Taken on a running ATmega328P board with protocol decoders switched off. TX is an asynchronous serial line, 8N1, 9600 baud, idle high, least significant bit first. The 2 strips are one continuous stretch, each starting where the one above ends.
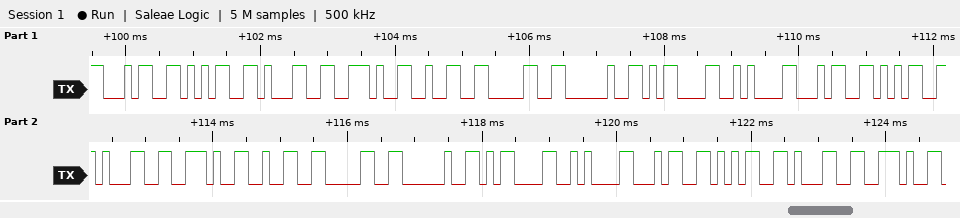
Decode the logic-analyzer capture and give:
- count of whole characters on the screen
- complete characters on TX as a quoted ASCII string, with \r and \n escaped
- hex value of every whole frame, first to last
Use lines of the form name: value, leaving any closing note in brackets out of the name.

count of whole characters on the screen: 22
complete characters on TX as a quoted ASCII string, with \r and \n escaped: "451.20 \r\n451.20 \r\n451."
hex value of every whole frame, first to last: 34 35 31 2E 32 30 20 0D 0A 34 35 31 2E 32 30 20 0D 0A 34 35 31 2E
